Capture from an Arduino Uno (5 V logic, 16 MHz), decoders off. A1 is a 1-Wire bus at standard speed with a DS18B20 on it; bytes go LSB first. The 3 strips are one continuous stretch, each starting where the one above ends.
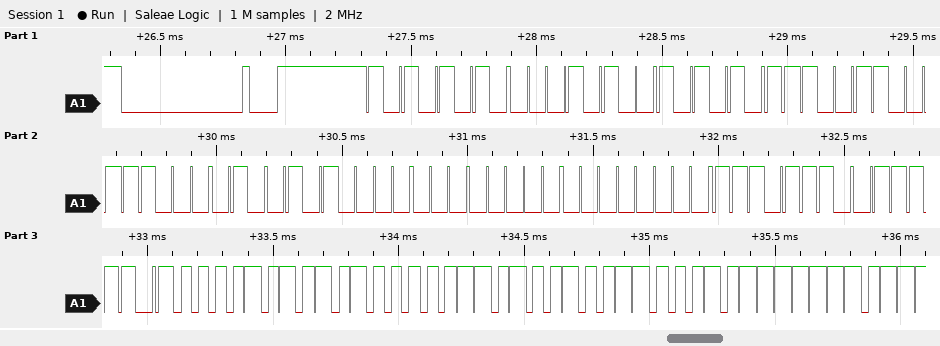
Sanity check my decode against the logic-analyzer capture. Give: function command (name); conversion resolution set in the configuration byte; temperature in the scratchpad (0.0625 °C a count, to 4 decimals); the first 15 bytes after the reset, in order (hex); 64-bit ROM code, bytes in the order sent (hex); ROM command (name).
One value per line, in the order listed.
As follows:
Read Scratchpad
12 bits
85.0000 °C
55 28 D5 99 43 0A 00 00 77 BE 50 05 4B 46 7F
28 D5 99 43 0A 00 00 77
Match ROM
